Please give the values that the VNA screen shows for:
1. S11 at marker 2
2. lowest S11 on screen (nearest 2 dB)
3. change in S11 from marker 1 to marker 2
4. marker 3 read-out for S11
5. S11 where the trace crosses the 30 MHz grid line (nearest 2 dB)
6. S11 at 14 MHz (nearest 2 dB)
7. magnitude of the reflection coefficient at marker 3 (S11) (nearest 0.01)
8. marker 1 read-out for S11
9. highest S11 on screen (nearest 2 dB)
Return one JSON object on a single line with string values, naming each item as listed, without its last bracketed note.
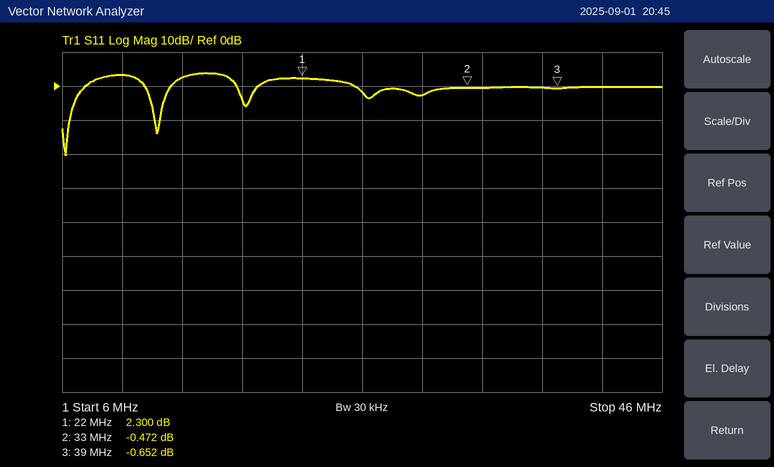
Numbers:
{"S11 at marker 2": "-0.472 dB", "lowest S11 on screen": "-20 dB", "change in S11 from marker 1 to marker 2": "-2.772 dB", "marker 3 read-out for S11": "-0.652 dB", "S11 where the trace crosses the 30 MHz grid line": "-2 dB", "S11 at 14 MHz": "2 dB", "magnitude of the reflection coefficient at marker 3 (S11)": "0.93", "marker 1 read-out for S11": "2.300 dB", "highest S11 on screen": "4 dB"}
